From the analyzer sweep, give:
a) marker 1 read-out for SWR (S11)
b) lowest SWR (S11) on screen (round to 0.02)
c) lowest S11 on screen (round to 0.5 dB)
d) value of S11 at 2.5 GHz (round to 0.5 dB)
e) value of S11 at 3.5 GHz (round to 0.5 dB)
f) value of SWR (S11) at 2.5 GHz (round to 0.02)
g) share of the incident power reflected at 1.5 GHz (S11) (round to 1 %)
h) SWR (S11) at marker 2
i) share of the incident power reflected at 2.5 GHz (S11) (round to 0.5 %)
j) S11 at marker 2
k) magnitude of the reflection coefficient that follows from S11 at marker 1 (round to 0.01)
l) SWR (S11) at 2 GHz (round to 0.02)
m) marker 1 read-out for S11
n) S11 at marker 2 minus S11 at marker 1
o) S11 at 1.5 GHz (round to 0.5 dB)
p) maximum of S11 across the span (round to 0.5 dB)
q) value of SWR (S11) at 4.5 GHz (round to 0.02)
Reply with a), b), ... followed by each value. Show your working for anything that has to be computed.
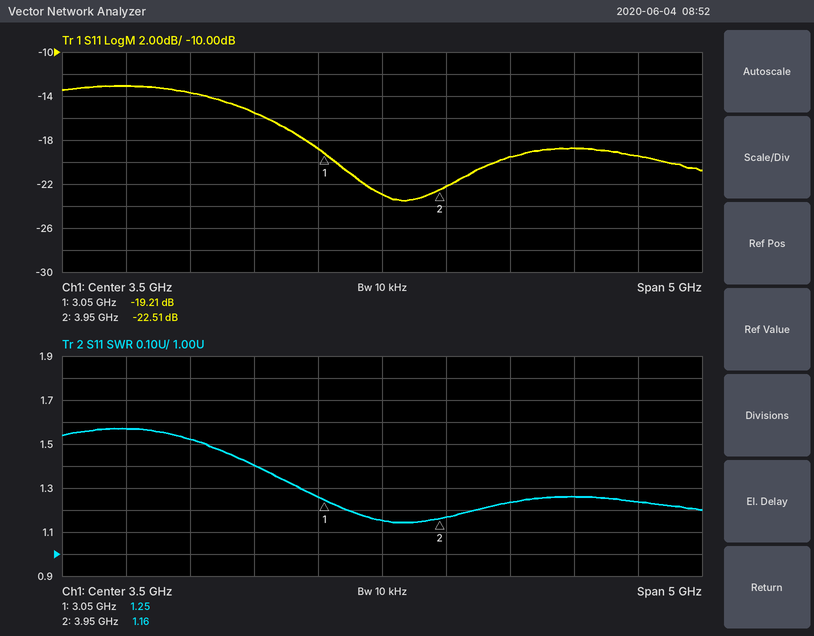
a) 1.25
b) 1.14
c) -23.5 dB
d) -15.5 dB
e) -23.0 dB
f) 1.40
g) 10^(-13/10) ≈ 5 %
h) 1.16
i) 10^(-15.5/10) ≈ 2.82 %, so 3.0 % to the nearest 0.5 %
j) -22.51 dB
k) 10^(-19.21/20) ≈ 0.11
l) 1.52
m) -19.21 dB
n) -22.51 − (-19.21) = -3.30 dB
o) -13.0 dB
p) -13.0 dB
q) 1.24
